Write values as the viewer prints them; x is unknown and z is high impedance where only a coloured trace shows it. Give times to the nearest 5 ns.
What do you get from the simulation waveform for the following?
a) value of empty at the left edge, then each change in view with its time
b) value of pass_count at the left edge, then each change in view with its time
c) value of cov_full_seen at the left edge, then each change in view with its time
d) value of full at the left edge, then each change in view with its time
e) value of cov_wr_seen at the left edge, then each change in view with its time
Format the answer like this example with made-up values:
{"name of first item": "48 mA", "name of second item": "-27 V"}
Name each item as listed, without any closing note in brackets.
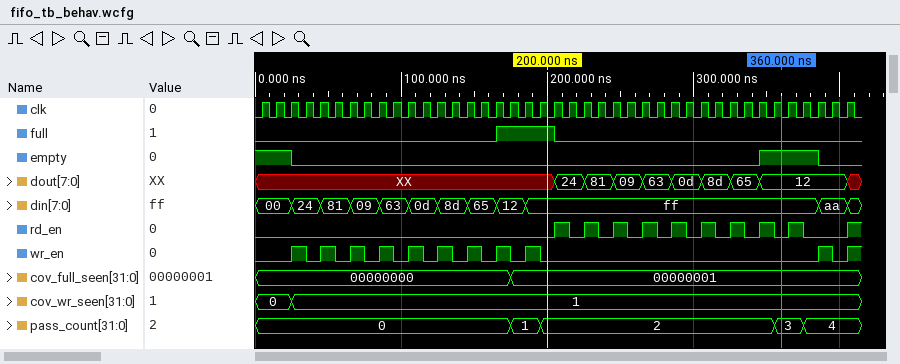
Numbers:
{"value of empty at the left edge, then each change in view with its time": "1, 0 at 25 ns, 1 at 345 ns, 0 at 385 ns", "value of pass_count at the left edge, then each change in view with its time": "0, 1 at 175 ns, 2 at 195 ns, 3 at 355 ns, 4 at 375 ns", "value of cov_full_seen at the left edge, then each change in view with its time": "00000000, 00000001 at 175 ns", "value of full at the left edge, then each change in view with its time": "0, 1 at 165 ns, 0 at 205 ns", "value of cov_wr_seen at the left edge, then each change in view with its time": "0, 1 at 25 ns"}
